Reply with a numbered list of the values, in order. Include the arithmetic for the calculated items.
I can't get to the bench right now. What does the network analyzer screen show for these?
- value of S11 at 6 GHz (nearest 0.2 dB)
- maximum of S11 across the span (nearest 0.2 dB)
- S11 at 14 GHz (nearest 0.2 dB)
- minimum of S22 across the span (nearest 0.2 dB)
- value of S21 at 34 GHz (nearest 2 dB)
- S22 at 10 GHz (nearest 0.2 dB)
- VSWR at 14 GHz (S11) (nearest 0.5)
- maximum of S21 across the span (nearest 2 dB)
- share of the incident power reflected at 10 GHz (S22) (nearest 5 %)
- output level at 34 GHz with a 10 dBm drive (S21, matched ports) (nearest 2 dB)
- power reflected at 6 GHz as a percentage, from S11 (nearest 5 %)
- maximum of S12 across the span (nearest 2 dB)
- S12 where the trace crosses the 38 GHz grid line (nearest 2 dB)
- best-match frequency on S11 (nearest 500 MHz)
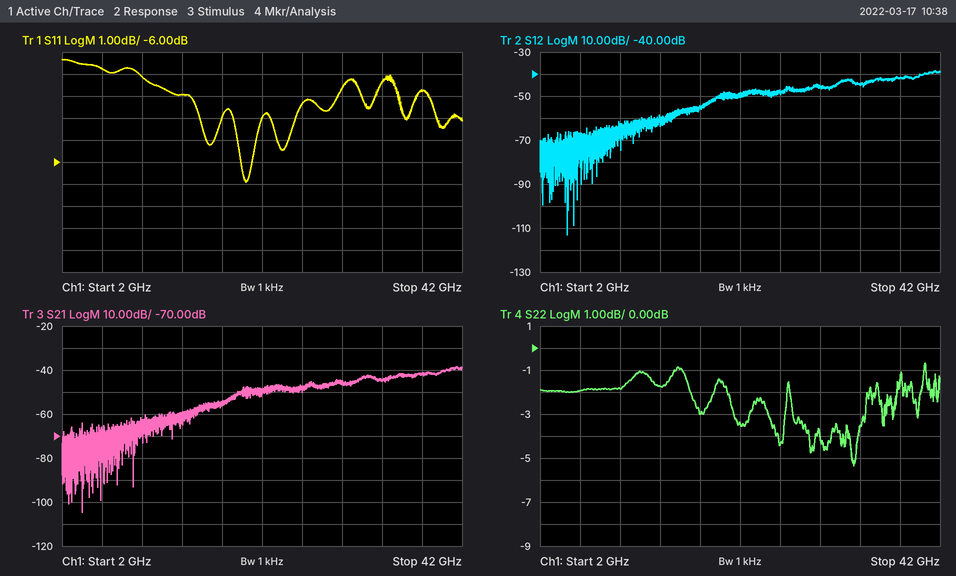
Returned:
1. -1.8 dB
2. -1.4 dB
3. -3.0 dB
4. -5.4 dB
5. -44 dB
6. -1.8 dB
7. |Γ| = 10^(-3/20) = 0.7079; VSWR = (1 + 0.7079)/(1 − 0.7079) ≈ 5.85, so 6.0 to the nearest 0.5
8. -38 dB
9. 10^(-1.8/10) ≈ 66.1 %, so 65 % to the nearest 5 %
10. 10 dBm + (-44 dB) = -34 dBm
11. 10^(-1.8/10) ≈ 66.1 %, so 65 % to the nearest 5 %
12. -38 dB
13. -42 dB
14. 20.5 GHz
